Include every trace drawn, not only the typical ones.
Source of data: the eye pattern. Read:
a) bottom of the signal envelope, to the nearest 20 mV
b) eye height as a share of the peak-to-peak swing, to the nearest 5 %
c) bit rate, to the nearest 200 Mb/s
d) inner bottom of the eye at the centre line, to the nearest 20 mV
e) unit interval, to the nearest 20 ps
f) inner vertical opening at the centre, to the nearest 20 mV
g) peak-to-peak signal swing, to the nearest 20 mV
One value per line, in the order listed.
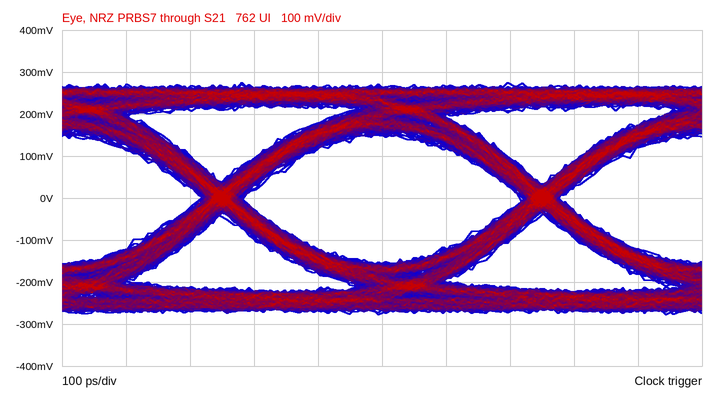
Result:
-280 mV
55 %
2.0 Gb/s
-160 mV
500 ps
300 mV
560 mV
